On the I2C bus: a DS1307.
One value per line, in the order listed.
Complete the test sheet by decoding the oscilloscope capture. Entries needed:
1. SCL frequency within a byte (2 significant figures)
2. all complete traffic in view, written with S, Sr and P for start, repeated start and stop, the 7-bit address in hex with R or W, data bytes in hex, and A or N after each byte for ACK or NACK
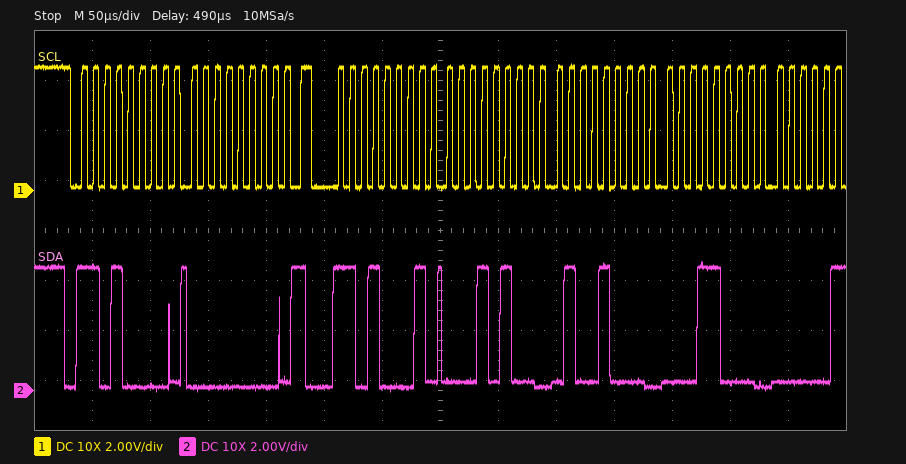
100 kHz
S 68W A 00 A Sr 68R A 14 A 48 A 18 A
